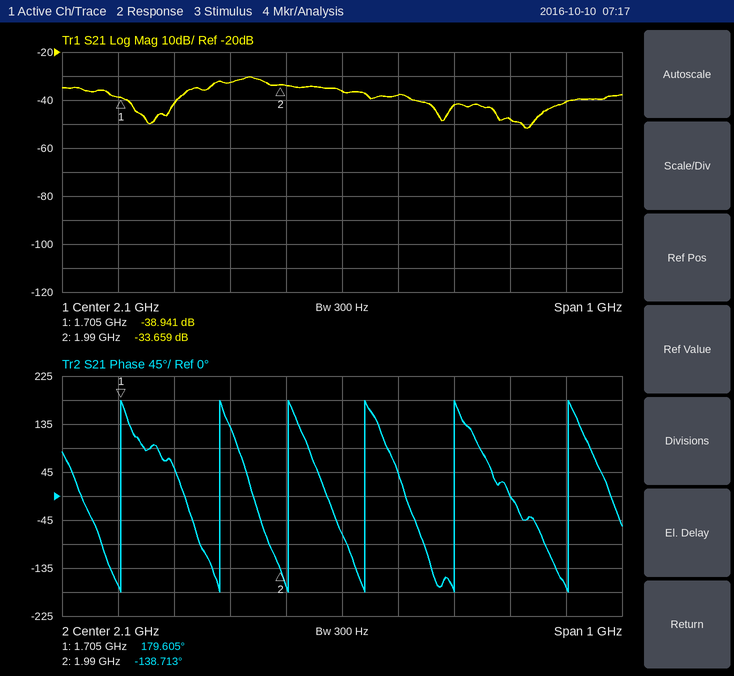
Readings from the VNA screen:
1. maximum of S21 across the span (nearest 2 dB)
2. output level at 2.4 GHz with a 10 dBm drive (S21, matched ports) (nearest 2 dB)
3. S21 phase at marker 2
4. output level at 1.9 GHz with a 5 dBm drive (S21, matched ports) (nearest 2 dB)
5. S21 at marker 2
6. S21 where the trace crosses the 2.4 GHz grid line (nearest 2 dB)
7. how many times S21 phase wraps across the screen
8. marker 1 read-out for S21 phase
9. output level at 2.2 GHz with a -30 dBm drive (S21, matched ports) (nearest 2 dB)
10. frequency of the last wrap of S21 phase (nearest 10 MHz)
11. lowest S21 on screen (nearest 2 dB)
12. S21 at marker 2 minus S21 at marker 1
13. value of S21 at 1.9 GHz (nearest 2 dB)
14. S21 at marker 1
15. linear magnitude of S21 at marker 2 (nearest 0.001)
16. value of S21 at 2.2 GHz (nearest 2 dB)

-30 dB
-38 dBm
-138.713°
-28 dBm
-33.659 dB
-48 dB
6
179.605°
-68 dBm
2.50 GHz
-52 dB
5.282 dB
-32 dB
-38.941 dB
0.021
-38 dB
